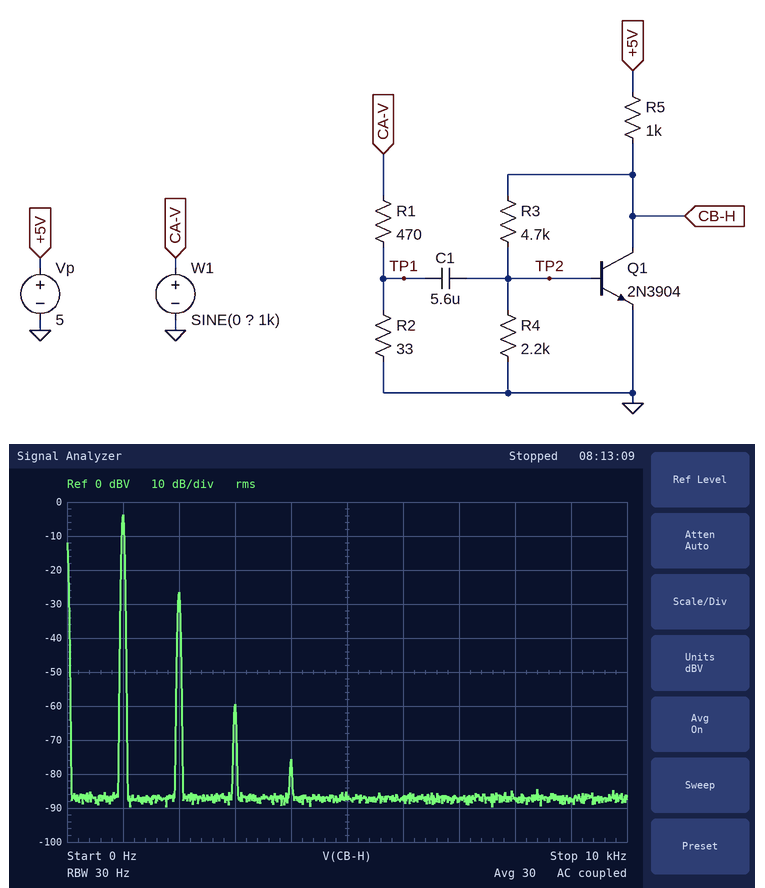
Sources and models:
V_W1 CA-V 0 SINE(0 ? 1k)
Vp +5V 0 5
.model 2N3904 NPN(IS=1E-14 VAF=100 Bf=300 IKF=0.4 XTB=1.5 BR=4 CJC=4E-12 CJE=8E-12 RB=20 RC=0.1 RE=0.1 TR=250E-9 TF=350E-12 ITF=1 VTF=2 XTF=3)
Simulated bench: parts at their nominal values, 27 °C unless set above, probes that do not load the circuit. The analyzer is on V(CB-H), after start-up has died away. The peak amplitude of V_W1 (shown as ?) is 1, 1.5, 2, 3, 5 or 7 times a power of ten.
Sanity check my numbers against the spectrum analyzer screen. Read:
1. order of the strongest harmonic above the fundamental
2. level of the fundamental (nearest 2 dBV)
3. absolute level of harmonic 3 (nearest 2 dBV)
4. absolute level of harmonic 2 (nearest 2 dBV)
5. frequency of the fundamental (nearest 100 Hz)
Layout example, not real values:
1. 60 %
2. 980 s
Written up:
1. 2
2. -4 dBV
3. -60 dBV
4. -26 dBV
5. 1.0 kHz
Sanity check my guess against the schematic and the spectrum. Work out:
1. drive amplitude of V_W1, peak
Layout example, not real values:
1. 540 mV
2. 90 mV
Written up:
1. 300 mV
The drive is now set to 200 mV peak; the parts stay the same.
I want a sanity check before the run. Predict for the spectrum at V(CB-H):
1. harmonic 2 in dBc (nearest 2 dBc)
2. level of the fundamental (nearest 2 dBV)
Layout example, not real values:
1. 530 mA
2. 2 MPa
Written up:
1. -26 dBc
2. -8 dBV
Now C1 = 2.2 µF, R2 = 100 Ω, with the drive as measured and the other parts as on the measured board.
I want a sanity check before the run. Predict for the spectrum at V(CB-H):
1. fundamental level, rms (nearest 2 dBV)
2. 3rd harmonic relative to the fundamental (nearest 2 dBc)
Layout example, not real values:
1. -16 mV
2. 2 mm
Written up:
1. 0 dBV
2. -42 dBc
